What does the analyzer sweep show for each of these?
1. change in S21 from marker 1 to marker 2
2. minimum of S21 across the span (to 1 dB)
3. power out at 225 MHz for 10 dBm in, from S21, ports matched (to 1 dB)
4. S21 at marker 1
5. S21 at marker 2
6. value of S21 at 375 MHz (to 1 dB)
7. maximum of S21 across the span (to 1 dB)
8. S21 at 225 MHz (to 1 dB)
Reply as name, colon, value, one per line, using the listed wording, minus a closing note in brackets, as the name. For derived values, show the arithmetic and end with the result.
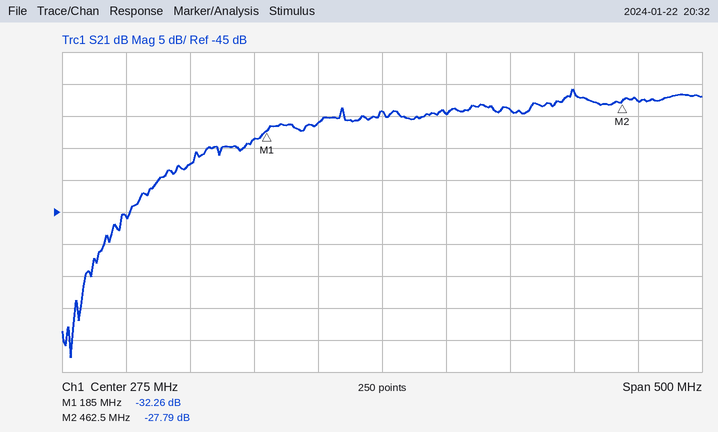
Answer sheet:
change in S21 from marker 1 to marker 2: -27.79 − (-32.26) = 4.47 dB
minimum of S21 across the span: -68 dB
power out at 225 MHz for 10 dBm in, from S21, ports matched: 10 dBm + (-31 dB) = -21 dBm
S21 at marker 1: -32.26 dB
S21 at marker 2: -27.79 dB
value of S21 at 375 MHz: -29 dB
maximum of S21 across the span: -26 dB
S21 at 225 MHz: -31 dB
